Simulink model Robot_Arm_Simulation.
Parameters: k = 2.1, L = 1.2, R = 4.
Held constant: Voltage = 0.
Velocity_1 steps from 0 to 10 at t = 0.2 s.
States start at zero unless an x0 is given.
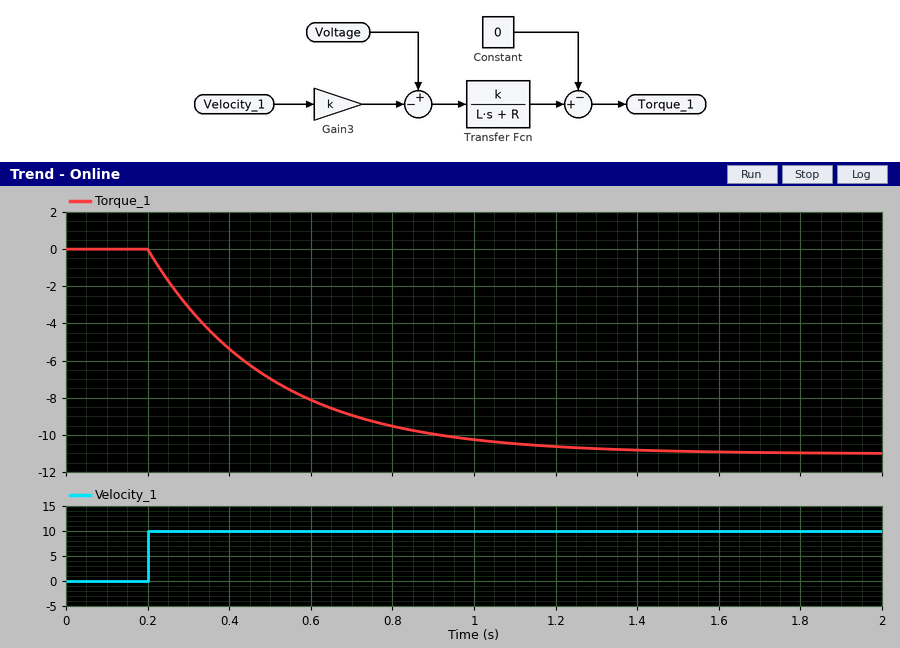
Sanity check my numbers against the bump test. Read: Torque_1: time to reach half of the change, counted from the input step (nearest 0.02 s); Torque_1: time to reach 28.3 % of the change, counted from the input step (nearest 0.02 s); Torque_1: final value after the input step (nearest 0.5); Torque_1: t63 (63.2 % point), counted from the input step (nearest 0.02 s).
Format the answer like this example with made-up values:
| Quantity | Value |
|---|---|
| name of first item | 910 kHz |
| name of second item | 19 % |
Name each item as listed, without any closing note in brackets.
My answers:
| Quantity | Value |
|---|---|
| Torque_1: time to reach half of the change, counted from the input step | 0.20 s |
| Torque_1: time to reach 28.3 % of the change, counted from the input step | 0.10 s |
| Torque_1: final value after the input step | -11.0 |
| Torque_1: t63 (63.2 % point), counted from the input step | 0.30 s |
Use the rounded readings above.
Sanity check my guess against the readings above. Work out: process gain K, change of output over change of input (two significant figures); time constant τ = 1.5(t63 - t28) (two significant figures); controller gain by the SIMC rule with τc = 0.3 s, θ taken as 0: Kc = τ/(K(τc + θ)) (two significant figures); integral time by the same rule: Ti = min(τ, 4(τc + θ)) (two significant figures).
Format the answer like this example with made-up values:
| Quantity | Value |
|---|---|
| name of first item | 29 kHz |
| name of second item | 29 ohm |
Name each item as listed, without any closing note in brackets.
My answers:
| Quantity | Value |
|---|---|
| process gain K, change of output over change of input | -1.1 |
| time constant τ = 1.5(t63 - t28) | 0.30 s |
| controller gain by the SIMC rule with τc = 0.3 s, θ taken as 0: Kc = τ/(K(τc + θ)) | -0.91 |
| integral time by the same rule: Ti = min(τ, 4(τc + θ)) | 0.30 s |
